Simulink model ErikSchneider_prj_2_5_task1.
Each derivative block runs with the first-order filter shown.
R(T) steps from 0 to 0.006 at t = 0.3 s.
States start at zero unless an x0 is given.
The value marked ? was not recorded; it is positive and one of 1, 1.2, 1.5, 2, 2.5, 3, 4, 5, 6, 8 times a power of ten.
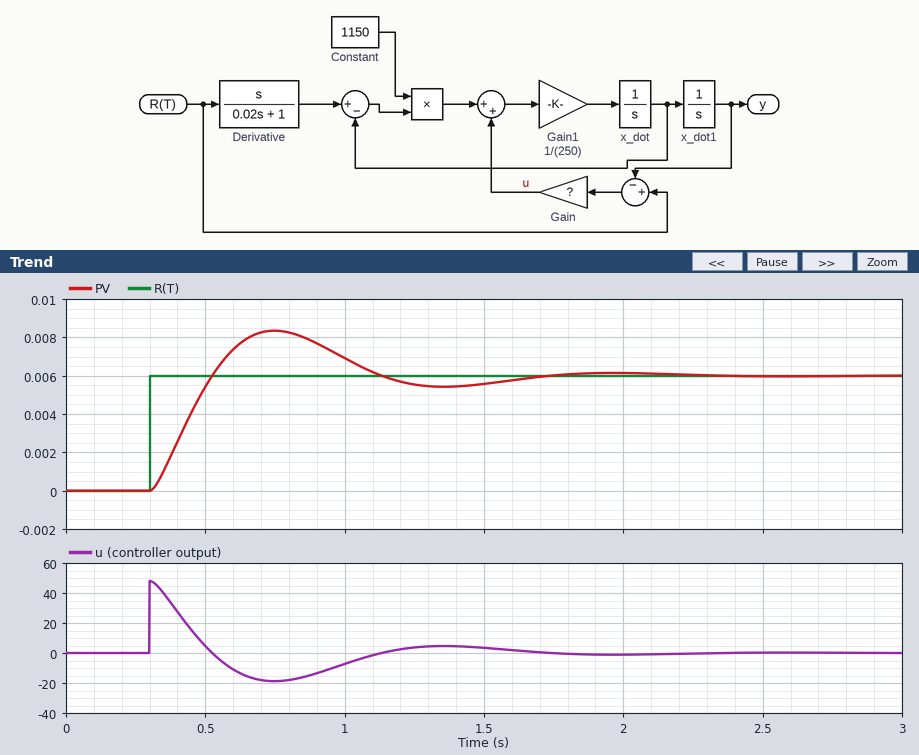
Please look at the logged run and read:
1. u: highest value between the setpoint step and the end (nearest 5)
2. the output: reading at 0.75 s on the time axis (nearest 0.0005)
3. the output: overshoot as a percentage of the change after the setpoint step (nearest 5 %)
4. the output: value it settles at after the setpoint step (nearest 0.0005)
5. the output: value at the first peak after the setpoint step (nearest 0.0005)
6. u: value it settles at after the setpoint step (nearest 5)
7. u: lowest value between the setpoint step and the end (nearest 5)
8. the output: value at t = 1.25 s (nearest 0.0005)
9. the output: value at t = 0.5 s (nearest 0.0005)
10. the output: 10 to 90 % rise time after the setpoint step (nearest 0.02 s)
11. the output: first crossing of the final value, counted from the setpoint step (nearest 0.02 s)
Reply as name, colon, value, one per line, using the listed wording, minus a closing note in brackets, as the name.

u: highest value between the setpoint step and the end: 50
the output: reading at 0.75 s on the time axis: 0.0085
the output: overshoot as a percentage of the change after the setpoint step: 40 %
the output: value it settles at after the setpoint step: 0.0060
the output: value at the first peak after the setpoint step: 0.0085
u: value it settles at after the setpoint step: 0
u: lowest value between the setpoint step and the end: -20
the output: value at t = 1.25 s: 0.0055
the output: value at t = 0.5 s: 0.0055
the output: 10 to 90 % rise time after the setpoint step: 0.16 s
the output: first crossing of the final value, counted from the setpoint step: 0.22 s
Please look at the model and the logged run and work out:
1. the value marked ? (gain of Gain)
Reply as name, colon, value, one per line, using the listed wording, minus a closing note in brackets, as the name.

the value marked ?: 8000
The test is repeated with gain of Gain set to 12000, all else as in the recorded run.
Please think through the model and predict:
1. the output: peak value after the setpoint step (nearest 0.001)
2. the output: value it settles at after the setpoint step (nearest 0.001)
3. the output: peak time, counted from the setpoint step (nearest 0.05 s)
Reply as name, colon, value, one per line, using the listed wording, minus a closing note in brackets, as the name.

the output: peak value after the setpoint step: 0.009
the output: value it settles at after the setpoint step: 0.006
the output: peak time, counted from the setpoint step: 0.40 s
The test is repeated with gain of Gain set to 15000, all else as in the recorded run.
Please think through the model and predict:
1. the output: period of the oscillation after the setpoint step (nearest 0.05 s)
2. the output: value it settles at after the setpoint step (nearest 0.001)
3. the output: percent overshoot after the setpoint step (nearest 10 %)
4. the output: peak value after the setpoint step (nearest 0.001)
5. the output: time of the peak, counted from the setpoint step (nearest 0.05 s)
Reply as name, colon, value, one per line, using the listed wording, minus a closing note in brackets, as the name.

the output: period of the oscillation after the setpoint step: 0.85 s
the output: value it settles at after the setpoint step: 0.006
the output: percent overshoot after the setpoint step: 50 %
the output: peak value after the setpoint step: 0.009
the output: time of the peak, counted from the setpoint step: 0.35 s
